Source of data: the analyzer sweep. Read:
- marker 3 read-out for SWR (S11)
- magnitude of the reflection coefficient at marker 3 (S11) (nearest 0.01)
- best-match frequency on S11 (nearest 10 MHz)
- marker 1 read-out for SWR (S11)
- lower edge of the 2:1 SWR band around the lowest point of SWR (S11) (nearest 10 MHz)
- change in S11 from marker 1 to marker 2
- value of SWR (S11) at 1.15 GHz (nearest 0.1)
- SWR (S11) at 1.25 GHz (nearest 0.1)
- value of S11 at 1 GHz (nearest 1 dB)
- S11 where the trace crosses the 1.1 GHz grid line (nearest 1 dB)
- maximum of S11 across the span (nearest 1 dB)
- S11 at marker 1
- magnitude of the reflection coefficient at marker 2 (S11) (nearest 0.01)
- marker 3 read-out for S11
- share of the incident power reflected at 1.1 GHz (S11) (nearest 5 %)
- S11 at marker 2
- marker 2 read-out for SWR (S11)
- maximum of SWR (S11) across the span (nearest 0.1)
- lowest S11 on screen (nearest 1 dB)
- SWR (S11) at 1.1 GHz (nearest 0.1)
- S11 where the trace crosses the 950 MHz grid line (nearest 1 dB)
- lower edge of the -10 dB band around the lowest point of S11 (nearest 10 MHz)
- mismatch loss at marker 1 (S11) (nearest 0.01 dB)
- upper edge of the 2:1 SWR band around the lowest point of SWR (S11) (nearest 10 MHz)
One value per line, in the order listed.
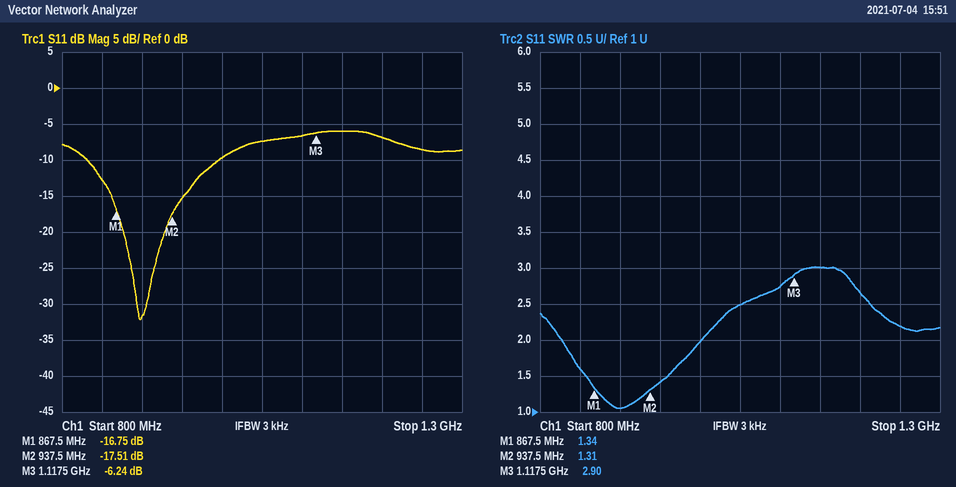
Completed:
2.90
0.49
900 MHz
1.34
830 MHz
-0.76 dB
3.0
2.2
-10 dB
-7 dB
-6 dB
-16.75 dB
0.13
-6.24 dB
20 %
-17.51 dB
1.31
3.0
-32 dB
2.7
-15 dB
830 MHz
0.09 dB
1.00 GHz
